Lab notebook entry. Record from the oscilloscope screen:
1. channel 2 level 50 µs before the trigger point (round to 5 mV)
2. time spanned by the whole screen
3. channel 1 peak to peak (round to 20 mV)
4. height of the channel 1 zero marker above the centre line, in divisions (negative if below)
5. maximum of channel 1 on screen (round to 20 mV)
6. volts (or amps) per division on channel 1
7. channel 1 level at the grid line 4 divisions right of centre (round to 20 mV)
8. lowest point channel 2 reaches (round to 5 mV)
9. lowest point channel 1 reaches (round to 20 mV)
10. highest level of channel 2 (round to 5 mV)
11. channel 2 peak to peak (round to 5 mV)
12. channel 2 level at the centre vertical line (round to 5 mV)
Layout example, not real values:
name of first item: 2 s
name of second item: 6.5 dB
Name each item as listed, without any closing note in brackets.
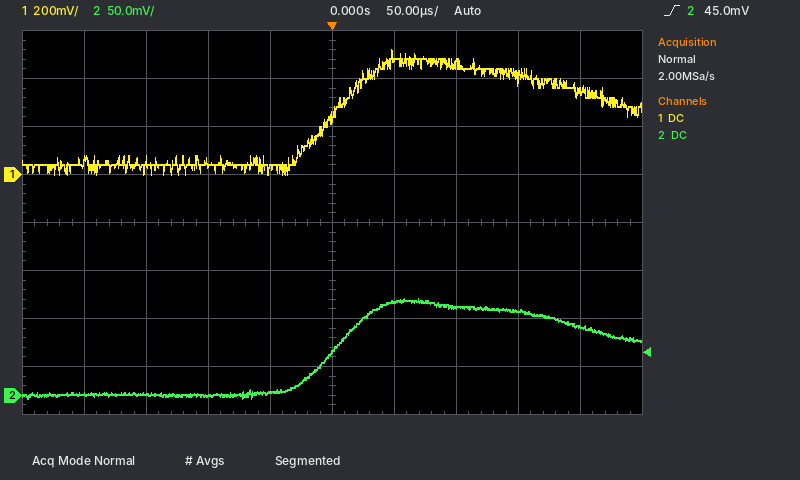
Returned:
channel 2 level 50 µs before the trigger point: 5 mV
time spanned by the whole screen: 500 µs
channel 1 peak to peak: 520 mV
height of the channel 1 zero marker above the centre line, in divisions: +1.0 div
maximum of channel 1 on screen: 520 mV
volts (or amps) per division on channel 1: 200 mV
channel 1 level at the grid line 4 divisions right of centre: 340 mV
lowest point channel 2 reaches: -5 mV
lowest point channel 1 reaches: 0 mV
highest level of channel 2: 100 mV
channel 2 peak to peak: 105 mV
channel 2 level at the centre vertical line: 45 mV
